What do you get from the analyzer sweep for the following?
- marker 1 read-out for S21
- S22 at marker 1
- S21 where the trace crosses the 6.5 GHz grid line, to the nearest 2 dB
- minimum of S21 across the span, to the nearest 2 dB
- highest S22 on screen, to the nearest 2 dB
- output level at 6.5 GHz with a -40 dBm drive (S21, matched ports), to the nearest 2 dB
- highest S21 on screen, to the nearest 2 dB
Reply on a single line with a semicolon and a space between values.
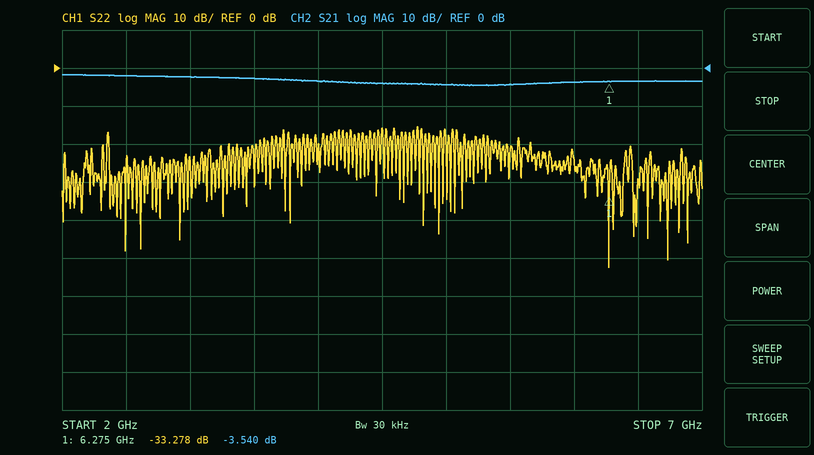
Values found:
-3.540 dB; -33.278 dB; -4 dB; -4 dB; -16 dB; -44 dBm; -2 dB
